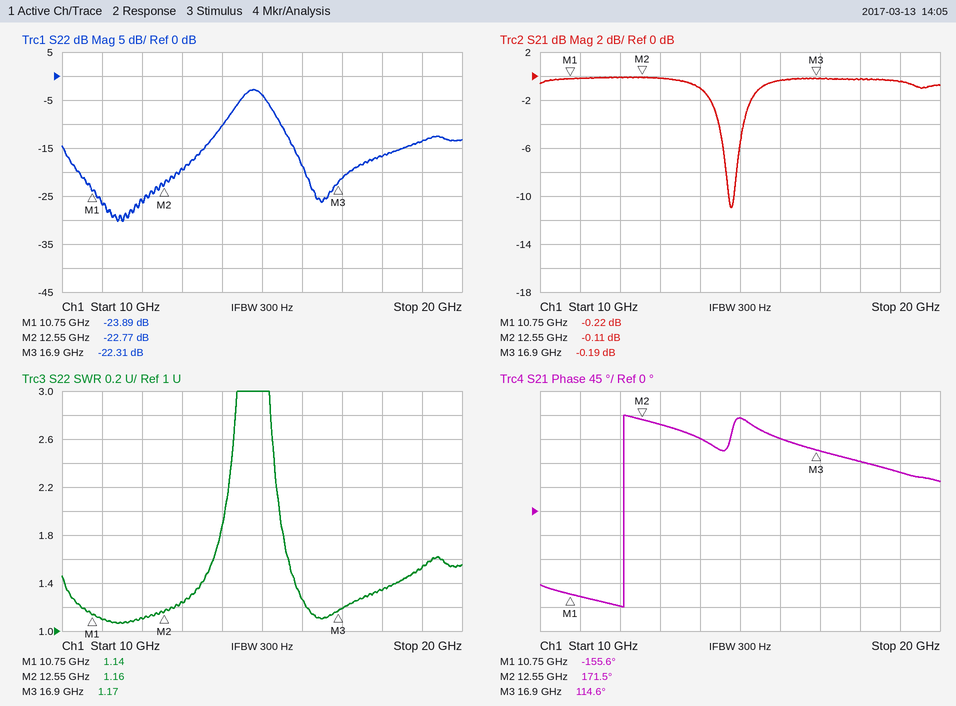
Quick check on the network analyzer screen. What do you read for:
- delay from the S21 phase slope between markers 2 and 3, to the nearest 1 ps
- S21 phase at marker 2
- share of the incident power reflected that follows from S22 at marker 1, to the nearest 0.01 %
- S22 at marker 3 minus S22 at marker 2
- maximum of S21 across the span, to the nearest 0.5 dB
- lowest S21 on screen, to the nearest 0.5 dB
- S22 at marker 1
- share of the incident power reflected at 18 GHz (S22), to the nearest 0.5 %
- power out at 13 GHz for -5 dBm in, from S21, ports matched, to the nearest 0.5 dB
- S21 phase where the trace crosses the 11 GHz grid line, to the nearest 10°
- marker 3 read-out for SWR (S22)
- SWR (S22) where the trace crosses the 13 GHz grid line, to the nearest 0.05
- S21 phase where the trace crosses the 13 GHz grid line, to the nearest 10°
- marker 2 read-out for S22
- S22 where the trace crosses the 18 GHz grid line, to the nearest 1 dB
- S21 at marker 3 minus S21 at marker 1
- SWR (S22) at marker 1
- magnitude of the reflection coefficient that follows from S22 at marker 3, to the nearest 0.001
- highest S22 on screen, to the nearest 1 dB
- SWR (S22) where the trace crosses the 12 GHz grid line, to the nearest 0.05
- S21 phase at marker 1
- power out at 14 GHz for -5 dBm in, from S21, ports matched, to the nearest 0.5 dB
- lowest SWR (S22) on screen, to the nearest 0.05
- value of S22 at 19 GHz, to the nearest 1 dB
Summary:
36 ps
171.5°
0.41 %
0.46 dB
0.0 dB
-11.0 dB
-23.89 dB
2.0 %
-5.0 dBm
-160°
1.17
1.25
160°
-22.77 dB
-17 dB
0.03 dB
1.14
0.077
-3 dB
1.10
-155.6°
-6.0 dBm
1.05
-14 dB
